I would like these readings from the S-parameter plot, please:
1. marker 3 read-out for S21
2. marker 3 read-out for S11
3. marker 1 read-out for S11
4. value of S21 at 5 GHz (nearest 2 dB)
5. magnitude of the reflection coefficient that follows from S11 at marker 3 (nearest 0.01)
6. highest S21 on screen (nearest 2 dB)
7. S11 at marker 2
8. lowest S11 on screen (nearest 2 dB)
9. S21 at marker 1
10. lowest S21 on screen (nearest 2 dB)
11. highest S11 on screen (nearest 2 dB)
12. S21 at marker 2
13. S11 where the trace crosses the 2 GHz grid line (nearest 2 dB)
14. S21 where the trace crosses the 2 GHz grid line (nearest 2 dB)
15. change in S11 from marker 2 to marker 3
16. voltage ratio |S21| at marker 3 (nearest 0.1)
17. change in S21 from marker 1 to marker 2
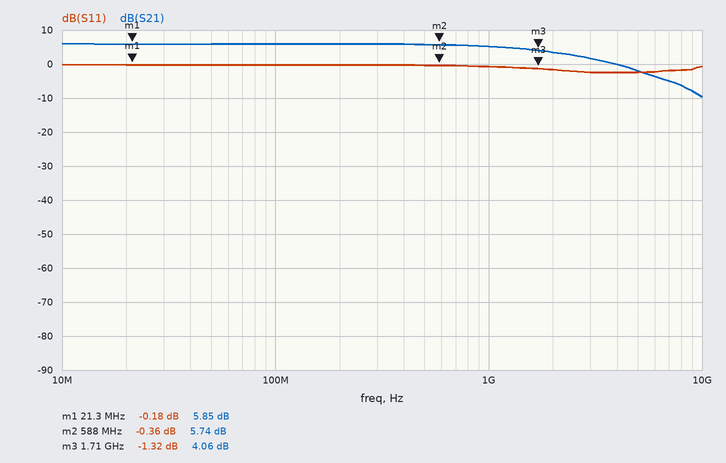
4.06 dB
-1.32 dB
-0.18 dB
-2 dB
0.86
6 dB
-0.36 dB
-2 dB
5.85 dB
-10 dB
0 dB
5.74 dB
-2 dB
4 dB
-0.96 dB
1.6
-0.11 dB
